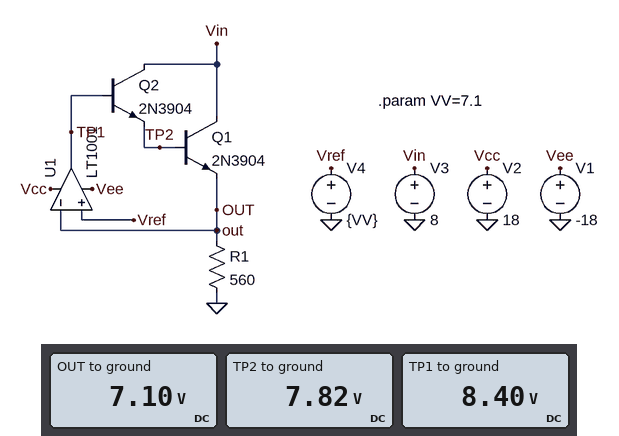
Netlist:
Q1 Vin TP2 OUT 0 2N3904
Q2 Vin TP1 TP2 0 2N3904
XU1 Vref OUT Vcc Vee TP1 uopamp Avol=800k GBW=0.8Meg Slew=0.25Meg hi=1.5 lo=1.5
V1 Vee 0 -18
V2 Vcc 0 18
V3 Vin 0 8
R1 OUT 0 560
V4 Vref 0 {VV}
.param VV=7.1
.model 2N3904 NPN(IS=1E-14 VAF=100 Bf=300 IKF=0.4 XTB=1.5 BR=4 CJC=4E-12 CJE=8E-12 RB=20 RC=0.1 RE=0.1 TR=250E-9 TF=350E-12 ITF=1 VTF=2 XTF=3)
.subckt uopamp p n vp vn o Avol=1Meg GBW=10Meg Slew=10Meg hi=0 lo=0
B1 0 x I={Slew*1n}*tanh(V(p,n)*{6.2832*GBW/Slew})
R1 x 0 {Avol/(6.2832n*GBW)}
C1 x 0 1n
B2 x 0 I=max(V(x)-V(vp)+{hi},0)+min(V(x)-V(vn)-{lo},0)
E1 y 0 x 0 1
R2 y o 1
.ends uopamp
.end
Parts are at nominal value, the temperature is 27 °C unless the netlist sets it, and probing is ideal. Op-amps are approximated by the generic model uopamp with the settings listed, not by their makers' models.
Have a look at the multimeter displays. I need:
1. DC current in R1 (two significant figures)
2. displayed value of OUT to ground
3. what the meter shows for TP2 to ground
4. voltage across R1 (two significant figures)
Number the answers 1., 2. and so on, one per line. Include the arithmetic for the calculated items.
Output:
1. (7.1 V) / 560 Ω = 13 mA
2. 7.10 V
3. 7.82 V
4. 7.1 V = 7.1 V
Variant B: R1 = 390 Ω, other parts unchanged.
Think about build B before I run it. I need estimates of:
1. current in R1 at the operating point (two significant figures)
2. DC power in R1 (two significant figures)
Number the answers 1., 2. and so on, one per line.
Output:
1. 18 mA
2. 130 mW
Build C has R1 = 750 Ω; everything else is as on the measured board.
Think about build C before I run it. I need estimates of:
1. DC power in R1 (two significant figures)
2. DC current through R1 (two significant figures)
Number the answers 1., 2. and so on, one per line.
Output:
1. 67 mW
2. 9.5 mA
